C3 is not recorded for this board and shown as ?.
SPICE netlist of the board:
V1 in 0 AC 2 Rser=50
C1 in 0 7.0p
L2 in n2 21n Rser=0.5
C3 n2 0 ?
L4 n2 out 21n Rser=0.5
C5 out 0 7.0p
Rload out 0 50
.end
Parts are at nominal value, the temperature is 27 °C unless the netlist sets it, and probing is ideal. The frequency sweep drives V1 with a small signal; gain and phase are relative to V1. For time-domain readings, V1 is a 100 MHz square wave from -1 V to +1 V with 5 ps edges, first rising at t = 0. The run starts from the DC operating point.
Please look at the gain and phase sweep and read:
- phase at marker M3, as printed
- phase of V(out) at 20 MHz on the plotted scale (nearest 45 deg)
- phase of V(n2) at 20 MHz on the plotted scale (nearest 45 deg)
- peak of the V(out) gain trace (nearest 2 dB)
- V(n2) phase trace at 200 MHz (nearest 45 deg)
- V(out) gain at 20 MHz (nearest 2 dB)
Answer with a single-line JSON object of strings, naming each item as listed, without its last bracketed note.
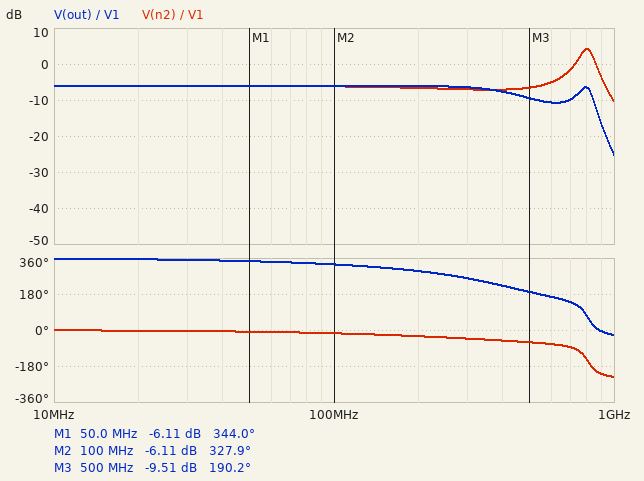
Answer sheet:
{"phase at marker M3, as printed": "190.2 deg", "phase of V(out) at 20 MHz on the plotted scale": "360 deg", "phase of V(n2) at 20 MHz on the plotted scale": "0 deg", "peak of the V(out) gain trace": "-6 dB", "V(n2) phase trace at 200 MHz": "-45 deg", "V(out) gain at 20 MHz": "-6 dB"}
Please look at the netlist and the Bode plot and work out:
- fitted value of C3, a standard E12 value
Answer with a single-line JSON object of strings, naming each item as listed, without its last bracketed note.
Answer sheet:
{"fitted value of C3, a standard E12 value": "4.7 pF"}
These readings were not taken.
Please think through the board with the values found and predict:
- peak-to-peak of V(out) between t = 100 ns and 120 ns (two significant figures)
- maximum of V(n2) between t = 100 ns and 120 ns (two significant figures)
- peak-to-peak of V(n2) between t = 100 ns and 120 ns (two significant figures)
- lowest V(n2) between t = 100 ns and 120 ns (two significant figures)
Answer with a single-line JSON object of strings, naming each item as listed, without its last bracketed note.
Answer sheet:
{"peak-to-peak of V(out) between t = 100 ns and 120 ns": "1.1 V", "maximum of V(n2) between t = 100 ns and 120 ns": "670 mV", "peak-to-peak of V(n2) between t = 100 ns and 120 ns": "1.3 V", "lowest V(n2) between t = 100 ns and 120 ns": "-670 mV"}
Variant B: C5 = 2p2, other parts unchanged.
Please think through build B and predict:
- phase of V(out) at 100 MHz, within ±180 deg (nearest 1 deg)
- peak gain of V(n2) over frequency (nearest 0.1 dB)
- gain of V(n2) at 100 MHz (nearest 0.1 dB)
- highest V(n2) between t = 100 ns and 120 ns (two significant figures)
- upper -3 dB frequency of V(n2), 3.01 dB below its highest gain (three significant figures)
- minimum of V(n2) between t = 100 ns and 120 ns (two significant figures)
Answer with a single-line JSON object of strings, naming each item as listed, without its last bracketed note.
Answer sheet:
{"phase of V(out) at 100 MHz, within ±180 deg": "-28 deg", "peak gain of V(n2) over frequency": "-0.9 dB", "gain of V(n2) at 100 MHz": "-5.9 dB", "highest V(n2) between t = 100 ns and 120 ns": "770 mV", "upper -3 dB frequency of V(n2), 3.01 dB below its highest gain": "867 MHz", "minimum of V(n2) between t = 100 ns and 120 ns": "-770 mV"}
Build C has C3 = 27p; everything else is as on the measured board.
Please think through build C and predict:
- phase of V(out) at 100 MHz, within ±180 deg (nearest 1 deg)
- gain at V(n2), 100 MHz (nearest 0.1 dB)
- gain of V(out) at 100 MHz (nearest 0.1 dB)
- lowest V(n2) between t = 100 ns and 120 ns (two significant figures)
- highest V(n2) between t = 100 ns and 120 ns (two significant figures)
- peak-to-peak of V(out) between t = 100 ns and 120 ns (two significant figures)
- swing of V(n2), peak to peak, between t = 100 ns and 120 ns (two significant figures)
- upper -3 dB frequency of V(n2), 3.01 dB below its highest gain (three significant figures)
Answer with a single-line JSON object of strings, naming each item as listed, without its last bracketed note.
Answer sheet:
{"phase of V(out) at 100 MHz, within ±180 deg": "-51 deg", "gain at V(n2), 100 MHz": "-6.7 dB", "gain of V(out) at 100 MHz": "-6.6 dB", "lowest V(n2) between t = 100 ns and 120 ns": "-510 mV", "highest V(n2) between t = 100 ns and 120 ns": "510 mV", "peak-to-peak of V(out) between t = 100 ns and 120 ns": "1.1 V", "swing of V(n2), peak to peak, between t = 100 ns and 120 ns": "1.0 V", "upper -3 dB frequency of V(n2), 3.01 dB below its highest gain": "442 MHz"}
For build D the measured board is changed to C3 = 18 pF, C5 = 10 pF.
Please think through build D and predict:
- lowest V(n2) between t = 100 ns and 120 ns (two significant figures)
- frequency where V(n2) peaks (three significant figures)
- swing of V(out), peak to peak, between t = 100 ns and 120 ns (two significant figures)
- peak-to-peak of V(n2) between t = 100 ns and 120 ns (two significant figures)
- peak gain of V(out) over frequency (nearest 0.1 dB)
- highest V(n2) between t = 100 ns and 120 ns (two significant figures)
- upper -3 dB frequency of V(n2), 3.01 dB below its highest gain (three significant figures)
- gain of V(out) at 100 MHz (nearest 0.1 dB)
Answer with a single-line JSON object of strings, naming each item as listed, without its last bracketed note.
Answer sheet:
{"lowest V(n2) between t = 100 ns and 120 ns": "-570 mV", "frequency where V(n2) peaks": "463 MHz", "swing of V(out), peak to peak, between t = 100 ns and 120 ns": "1.2 V", "peak-to-peak of V(n2) between t = 100 ns and 120 ns": "1.1 V", "peak gain of V(out) over frequency": "-6.1 dB", "highest V(n2) between t = 100 ns and 120 ns": "570 mV", "upper -3 dB frequency of V(n2), 3.01 dB below its highest gain": "543 MHz", "gain of V(out) at 100 MHz": "-6.4 dB"}
